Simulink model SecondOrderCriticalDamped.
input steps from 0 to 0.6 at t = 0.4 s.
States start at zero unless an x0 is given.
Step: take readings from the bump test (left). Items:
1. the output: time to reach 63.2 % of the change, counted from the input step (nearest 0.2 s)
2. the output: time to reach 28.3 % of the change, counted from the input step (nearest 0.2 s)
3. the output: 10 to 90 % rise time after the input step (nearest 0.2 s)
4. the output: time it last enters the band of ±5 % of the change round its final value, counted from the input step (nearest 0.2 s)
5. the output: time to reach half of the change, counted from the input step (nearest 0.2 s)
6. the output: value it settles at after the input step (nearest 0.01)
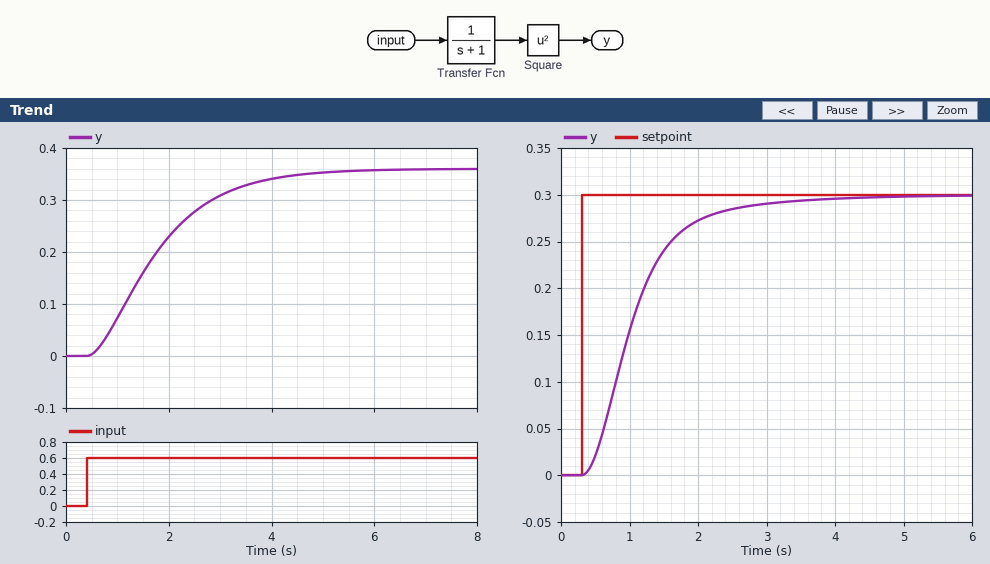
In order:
1.6 s
0.8 s
2.6 s
3.6 s
1.2 s
0.36
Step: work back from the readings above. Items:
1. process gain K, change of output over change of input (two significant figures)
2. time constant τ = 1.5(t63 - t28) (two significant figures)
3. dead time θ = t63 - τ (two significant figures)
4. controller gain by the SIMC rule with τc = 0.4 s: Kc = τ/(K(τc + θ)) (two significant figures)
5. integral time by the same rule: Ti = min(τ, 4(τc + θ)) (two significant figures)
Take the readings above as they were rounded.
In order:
0.60
1.2 s
0.40 s
2.5
1.2 s
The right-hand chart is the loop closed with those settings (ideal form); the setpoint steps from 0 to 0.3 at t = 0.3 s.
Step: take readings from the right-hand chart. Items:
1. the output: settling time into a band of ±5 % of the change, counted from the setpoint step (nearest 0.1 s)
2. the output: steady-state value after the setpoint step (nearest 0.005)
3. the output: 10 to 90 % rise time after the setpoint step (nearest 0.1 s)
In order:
2.2 s
0.300
1.4 s
